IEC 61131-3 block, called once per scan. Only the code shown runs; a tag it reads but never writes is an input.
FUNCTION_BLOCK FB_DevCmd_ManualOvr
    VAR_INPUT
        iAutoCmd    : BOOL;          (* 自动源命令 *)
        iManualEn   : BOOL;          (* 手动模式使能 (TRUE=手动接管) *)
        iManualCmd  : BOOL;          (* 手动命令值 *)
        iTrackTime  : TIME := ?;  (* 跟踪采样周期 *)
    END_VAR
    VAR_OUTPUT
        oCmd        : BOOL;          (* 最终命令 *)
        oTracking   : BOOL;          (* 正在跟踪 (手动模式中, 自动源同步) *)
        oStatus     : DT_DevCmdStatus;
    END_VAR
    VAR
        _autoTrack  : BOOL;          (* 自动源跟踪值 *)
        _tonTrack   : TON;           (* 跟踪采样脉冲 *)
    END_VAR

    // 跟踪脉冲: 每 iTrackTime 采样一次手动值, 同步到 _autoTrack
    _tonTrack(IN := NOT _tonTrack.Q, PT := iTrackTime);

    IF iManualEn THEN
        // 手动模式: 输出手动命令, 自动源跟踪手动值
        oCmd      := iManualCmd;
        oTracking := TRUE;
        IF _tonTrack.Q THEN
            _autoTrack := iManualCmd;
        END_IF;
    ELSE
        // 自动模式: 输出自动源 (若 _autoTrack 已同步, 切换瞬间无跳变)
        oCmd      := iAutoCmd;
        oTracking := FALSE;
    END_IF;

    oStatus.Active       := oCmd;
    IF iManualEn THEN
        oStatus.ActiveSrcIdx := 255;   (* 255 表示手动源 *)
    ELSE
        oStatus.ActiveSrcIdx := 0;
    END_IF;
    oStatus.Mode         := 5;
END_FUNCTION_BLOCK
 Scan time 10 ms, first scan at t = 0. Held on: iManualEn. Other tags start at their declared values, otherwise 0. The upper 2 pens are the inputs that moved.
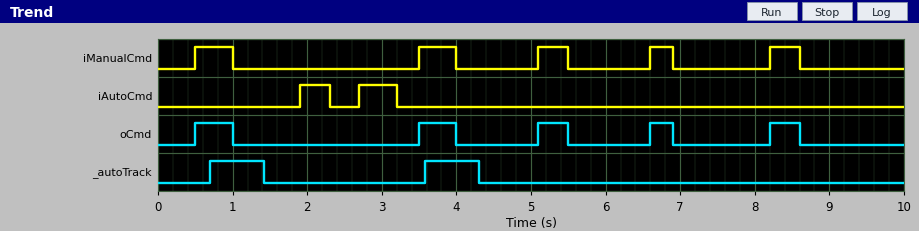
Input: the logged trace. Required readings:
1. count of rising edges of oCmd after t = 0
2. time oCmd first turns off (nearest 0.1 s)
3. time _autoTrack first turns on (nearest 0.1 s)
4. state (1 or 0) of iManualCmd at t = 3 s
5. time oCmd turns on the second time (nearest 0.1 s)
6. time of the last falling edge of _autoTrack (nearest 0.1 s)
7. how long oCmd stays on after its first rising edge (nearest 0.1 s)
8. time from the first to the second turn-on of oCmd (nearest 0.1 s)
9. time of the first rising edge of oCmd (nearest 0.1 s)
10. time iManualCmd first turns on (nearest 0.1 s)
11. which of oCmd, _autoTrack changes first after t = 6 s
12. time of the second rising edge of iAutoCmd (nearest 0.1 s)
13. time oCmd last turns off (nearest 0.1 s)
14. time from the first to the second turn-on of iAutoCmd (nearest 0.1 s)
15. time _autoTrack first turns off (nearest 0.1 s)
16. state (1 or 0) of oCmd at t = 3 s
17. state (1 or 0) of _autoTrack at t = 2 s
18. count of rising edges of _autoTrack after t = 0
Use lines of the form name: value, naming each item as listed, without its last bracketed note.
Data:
count of rising edges of oCmd after t = 0: 5
time oCmd first turns off: 1.0 s
time _autoTrack first turns on: 0.7 s
state (1 or 0) of iManualCmd at t = 3 s: 0
time oCmd turns on the second time: 3.5 s
time of the last falling edge of _autoTrack: 4.3 s
how long oCmd stays on after its first rising edge: 0.5 s
time from the first to the second turn-on of oCmd: 3.0 s
time of the first rising edge of oCmd: 0.5 s
time iManualCmd first turns on: 0.5 s
which of oCmd, _autoTrack changes first after t = 6 s: oCmd
time of the second rising edge of iAutoCmd: 2.7 s
time oCmd last turns off: 8.6 s
time from the first to the second turn-on of iAutoCmd: 0.8 s
time _autoTrack first turns off: 1.4 s
state (1 or 0) of oCmd at t = 3 s: 0
state (1 or 0) of _autoTrack at t = 2 s: 0
count of rising edges of _autoTrack after t = 0: 2
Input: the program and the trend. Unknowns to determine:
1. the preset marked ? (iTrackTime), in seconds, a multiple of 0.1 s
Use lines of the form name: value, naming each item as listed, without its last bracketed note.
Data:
the preset marked ? (iTrackTime), in seconds, a multiple of 0.1 s: 0.7 s
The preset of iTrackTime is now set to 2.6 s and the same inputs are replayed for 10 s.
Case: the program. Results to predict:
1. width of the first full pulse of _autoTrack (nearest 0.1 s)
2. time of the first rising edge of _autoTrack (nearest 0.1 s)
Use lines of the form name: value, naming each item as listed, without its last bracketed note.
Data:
width of the first full pulse of _autoTrack: 2.6 s
time of the first rising edge of _autoTrack: 5.2 s
